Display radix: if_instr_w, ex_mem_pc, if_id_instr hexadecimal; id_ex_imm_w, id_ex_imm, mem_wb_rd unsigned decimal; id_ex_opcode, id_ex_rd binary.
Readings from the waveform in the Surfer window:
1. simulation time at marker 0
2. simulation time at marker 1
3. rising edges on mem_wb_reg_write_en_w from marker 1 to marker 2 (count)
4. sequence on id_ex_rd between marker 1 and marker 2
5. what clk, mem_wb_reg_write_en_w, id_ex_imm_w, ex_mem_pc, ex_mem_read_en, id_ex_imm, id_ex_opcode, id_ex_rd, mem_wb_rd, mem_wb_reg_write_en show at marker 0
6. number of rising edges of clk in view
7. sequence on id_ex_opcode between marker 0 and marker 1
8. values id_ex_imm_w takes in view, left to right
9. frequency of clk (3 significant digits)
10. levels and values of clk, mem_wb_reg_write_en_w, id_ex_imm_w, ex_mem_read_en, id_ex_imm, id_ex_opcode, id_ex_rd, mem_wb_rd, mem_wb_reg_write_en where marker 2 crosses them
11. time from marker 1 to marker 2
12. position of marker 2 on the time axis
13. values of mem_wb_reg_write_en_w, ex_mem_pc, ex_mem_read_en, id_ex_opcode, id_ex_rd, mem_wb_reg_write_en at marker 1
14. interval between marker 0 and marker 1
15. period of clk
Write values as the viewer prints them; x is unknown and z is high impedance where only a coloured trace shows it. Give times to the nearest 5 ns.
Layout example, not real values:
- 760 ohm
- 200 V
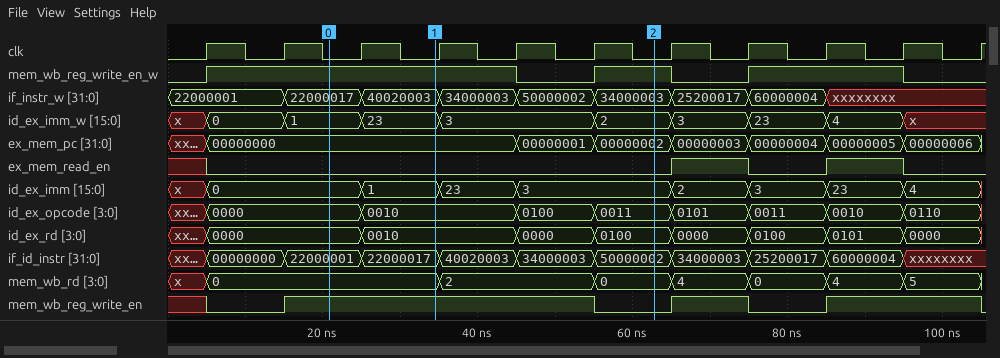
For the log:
- 20 ns
- 35 ns
- 1
- 0010, 0000, 0100
- clk=0, mem_wb_reg_write_en_w=1, id_ex_imm_w=1, ex_mem_pc=00000000, ex_mem_read_en=0, id_ex_imm=0, id_ex_opcode=0000, id_ex_rd=0000, mem_wb_rd=0, mem_wb_reg_write_en=1
- 11
- 0000, 0010
- x, 0, 1, 23, 3, 2, 3, 23, 4, x
- 100 MHz
- clk=0, mem_wb_reg_write_en_w=1, id_ex_imm_w=2, ex_mem_read_en=0, id_ex_imm=3, id_ex_opcode=0011, id_ex_rd=0100, mem_wb_rd=0, mem_wb_reg_write_en=0
- 30 ns
- 65 ns
- mem_wb_reg_write_en_w=1, ex_mem_pc=00000000, ex_mem_read_en=0, id_ex_opcode=0010, id_ex_rd=0010, mem_wb_reg_write_en=1
- 15 ns
- 10 ns
